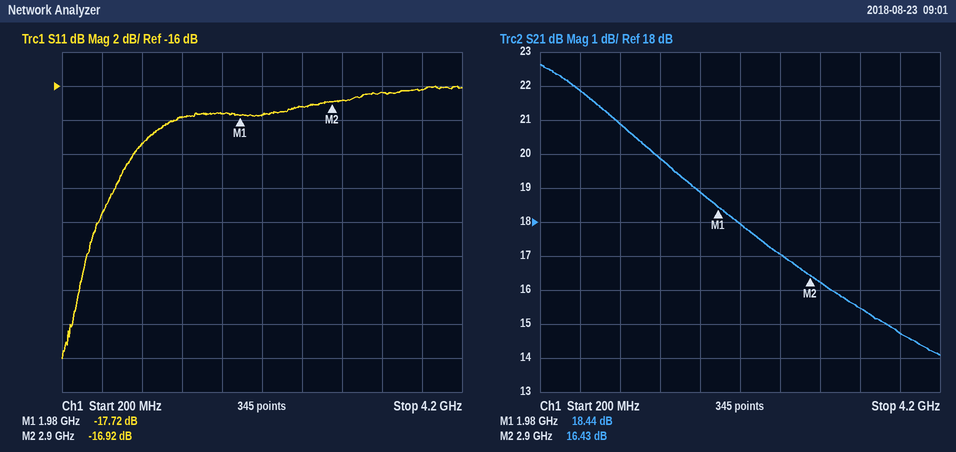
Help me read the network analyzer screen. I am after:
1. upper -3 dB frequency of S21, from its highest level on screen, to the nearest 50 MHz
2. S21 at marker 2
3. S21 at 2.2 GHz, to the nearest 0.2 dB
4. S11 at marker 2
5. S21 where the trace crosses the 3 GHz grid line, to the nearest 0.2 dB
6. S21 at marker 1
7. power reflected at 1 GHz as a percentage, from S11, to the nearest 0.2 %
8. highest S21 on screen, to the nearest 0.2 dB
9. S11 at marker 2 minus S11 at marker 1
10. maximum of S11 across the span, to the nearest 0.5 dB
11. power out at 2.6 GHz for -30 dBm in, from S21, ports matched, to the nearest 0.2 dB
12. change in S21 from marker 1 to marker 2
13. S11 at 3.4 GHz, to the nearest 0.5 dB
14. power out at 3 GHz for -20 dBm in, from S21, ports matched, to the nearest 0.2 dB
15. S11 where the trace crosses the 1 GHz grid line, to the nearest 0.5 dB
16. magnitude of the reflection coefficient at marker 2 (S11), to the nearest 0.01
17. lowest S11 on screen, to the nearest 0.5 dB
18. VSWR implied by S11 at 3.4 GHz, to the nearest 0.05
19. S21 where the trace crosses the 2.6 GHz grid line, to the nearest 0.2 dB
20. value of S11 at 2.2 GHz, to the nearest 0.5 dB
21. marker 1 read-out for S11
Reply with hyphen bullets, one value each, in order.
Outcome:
- 1.50 GHz
- 16.43 dB
- 18.0 dB
- -16.92 dB
- 16.2 dB
- 18.44 dB
- 1.2 %
- 22.6 dB
- 0.80 dB
- -16.0 dB
- -13.0 dBm
- -2.01 dB
- -16.5 dB
- -3.8 dBm
- -19.5 dB
- 0.14
- -32.0 dB
- 1.35
- 17.0 dB
- -17.5 dB
- -17.72 dB
